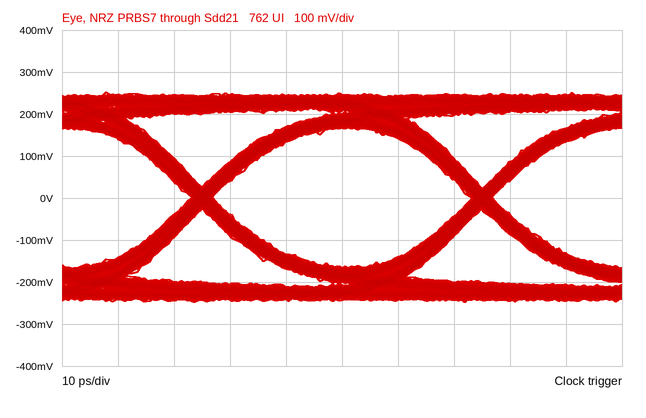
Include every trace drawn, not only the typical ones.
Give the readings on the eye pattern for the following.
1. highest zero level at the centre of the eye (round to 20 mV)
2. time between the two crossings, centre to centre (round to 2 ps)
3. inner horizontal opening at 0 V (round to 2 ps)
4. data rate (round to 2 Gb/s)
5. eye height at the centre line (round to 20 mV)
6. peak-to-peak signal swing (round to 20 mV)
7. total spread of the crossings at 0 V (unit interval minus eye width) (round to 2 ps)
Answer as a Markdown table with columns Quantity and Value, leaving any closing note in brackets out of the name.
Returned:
| Quantity | Value |
|---|---|
| highest zero level at the centre of the eye | -160 mV |
| time between the two crossings, centre to centre | 50 ps |
| inner horizontal opening at 0 V | 46 ps |
| data rate | 20 Gb/s |
| eye height at the centre line | 340 mV |
| peak-to-peak signal swing | 500 mV |
| total spread of the crossings at 0 V (unit interval minus eye width) | 4 ps |
